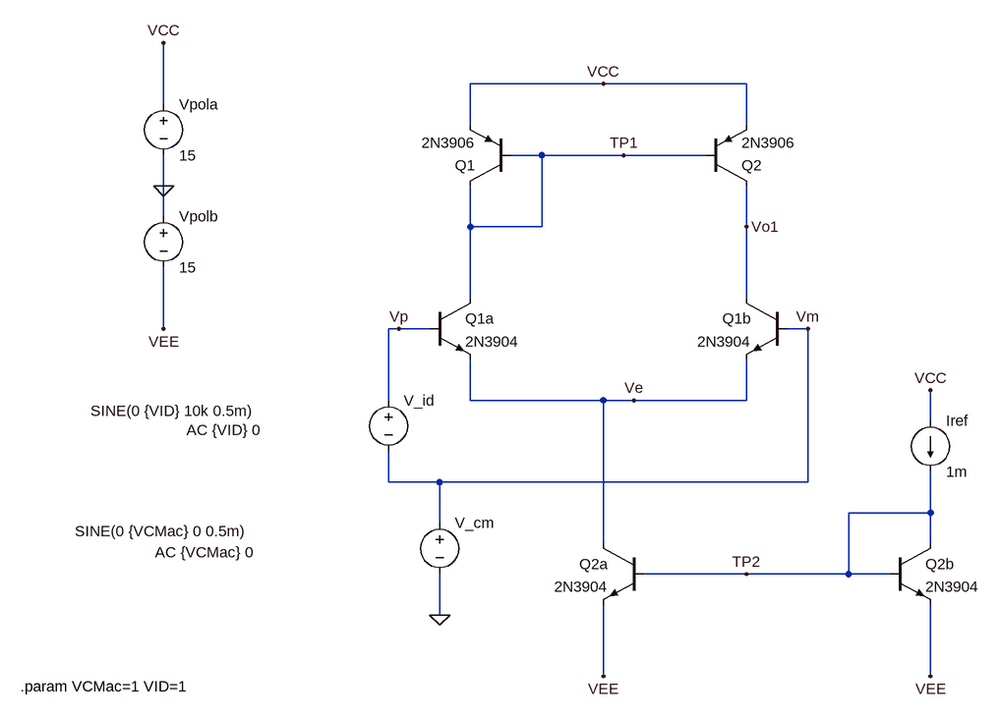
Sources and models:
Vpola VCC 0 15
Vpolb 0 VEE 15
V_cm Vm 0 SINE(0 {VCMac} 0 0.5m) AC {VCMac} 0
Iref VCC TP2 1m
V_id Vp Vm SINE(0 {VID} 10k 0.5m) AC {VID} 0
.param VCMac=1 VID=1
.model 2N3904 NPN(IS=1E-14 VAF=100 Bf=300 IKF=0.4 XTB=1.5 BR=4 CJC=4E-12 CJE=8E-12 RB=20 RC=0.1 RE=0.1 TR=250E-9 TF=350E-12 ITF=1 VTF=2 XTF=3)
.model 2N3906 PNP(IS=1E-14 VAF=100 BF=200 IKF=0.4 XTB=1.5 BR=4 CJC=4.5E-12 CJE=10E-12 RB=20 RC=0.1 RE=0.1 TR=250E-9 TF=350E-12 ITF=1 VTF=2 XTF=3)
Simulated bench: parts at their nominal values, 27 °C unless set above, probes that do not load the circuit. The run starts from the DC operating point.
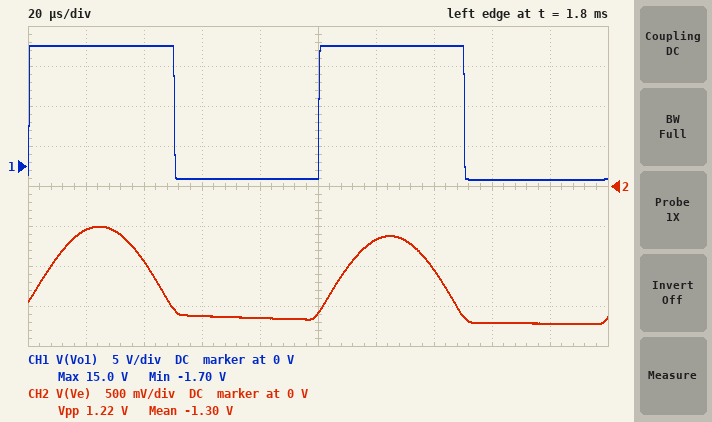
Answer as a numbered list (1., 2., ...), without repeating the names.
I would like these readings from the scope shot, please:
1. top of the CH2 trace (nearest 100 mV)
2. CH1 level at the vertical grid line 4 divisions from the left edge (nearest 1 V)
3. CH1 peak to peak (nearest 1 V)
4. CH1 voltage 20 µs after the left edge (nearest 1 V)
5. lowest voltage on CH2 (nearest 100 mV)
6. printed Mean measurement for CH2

1. -500 mV
2. -2 V
3. 17 V
4. 15 V
5. -1.7 V
6. -1.30 V
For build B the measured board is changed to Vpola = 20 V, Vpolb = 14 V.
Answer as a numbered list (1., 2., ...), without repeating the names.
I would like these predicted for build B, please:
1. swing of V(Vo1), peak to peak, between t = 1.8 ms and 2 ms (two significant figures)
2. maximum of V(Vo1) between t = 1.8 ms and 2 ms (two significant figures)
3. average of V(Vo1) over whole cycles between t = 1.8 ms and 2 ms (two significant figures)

1. 22 V
2. 20 V
3. 9.2 V
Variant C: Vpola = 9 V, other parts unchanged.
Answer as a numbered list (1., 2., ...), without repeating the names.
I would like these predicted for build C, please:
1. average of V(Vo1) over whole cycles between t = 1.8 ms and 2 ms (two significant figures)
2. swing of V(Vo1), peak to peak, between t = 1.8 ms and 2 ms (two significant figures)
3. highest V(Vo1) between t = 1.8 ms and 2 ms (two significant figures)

1. 3.7 V
2. 11 V
3. 9.0 V
